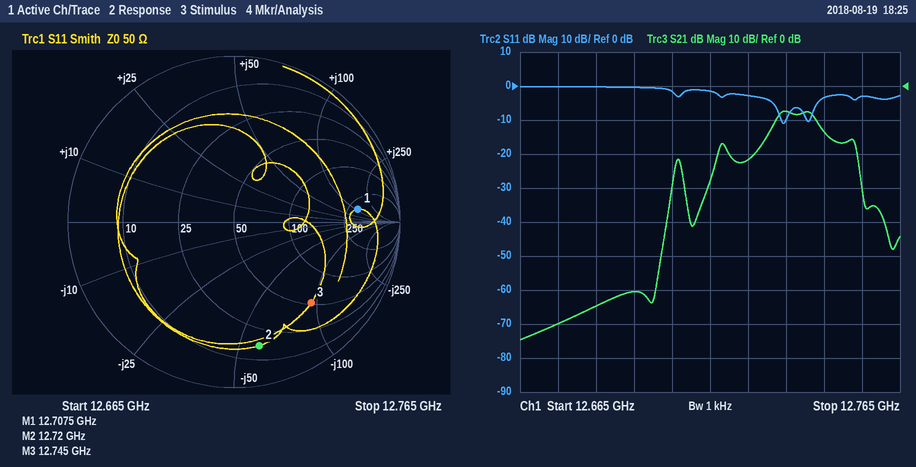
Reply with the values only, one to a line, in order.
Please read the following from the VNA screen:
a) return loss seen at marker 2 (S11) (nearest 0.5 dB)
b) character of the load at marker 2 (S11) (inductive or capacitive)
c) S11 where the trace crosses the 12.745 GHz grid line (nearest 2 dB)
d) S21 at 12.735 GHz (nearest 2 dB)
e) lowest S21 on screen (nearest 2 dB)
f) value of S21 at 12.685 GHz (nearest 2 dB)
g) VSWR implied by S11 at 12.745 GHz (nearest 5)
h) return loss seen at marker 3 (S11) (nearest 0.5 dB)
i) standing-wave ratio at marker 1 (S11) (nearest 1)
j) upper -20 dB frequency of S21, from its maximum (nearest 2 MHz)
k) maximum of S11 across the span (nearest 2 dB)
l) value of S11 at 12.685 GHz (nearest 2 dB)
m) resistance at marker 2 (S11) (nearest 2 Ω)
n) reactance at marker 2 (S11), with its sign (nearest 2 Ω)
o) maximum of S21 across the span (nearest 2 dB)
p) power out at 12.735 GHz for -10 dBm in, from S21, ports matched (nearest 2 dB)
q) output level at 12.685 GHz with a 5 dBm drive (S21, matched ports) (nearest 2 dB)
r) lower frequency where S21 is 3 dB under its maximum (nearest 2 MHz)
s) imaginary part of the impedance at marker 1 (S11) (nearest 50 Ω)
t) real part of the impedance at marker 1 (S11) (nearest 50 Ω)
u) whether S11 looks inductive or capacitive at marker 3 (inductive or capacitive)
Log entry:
2.5 dB
capacitive
-4 dB
-8 dB
-74 dB
-64 dB
5
3.5 dB
7
12.754 GHz
0 dB
0 dB
16 Ω
-58 Ω
-8 dB
-18 dBm
-60 dBm
12.732 GHz
+100 Ω
300 Ω
capacitive
